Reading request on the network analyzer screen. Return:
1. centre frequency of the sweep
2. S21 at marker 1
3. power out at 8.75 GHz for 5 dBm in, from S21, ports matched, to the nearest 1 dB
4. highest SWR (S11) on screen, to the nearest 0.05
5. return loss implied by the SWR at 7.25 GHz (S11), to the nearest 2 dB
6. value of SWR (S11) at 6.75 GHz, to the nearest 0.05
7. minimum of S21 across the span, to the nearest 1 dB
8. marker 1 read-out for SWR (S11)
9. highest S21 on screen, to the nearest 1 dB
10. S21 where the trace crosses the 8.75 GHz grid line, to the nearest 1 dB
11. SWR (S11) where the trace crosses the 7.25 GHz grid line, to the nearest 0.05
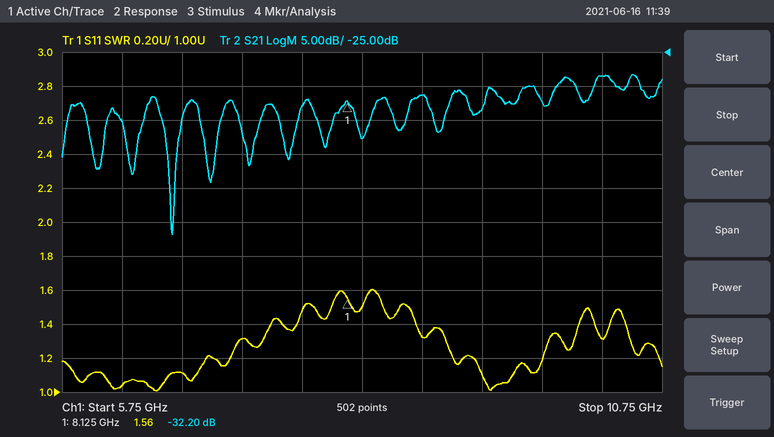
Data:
8.25 GHz
-32.20 dB
-26 dBm
1.60
18 dB
1.10
-52 dB
1.56
-28 dB
-31 dB
1.30
